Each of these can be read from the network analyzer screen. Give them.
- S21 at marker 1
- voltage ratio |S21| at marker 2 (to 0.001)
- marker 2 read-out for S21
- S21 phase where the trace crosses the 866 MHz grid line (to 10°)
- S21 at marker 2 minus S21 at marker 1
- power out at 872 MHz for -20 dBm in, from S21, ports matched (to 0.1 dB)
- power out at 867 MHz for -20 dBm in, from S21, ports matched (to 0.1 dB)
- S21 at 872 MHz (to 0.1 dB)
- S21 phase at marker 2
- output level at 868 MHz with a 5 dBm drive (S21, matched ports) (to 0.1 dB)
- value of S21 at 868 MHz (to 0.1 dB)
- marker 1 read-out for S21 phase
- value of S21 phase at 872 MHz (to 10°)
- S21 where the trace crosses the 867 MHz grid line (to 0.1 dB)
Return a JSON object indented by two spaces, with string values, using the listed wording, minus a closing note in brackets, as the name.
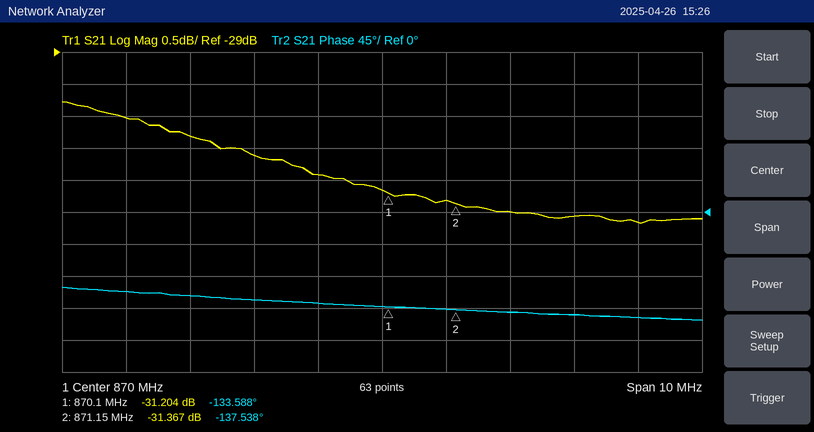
{
  "S21 at marker 1": "-31.204 dB",
  "voltage ratio |S21| at marker 2": "0.027",
  "marker 2 read-out for S21": "-31.367 dB",
  "S21 phase where the trace crosses the 866 MHz grid line": "-110°",
  "S21 at marker 2 minus S21 at marker 1": "-0.163 dB",
  "power out at 872 MHz for -20 dBm in, from S21, ports matched": "-51.5 dBm",
  "power out at 867 MHz for -20 dBm in, from S21, ports matched": "-50.3 dBm",
  "S21 at 872 MHz": "-31.5 dB",
  "S21 phase at marker 2": "-137.538°",
  "output level at 868 MHz with a 5 dBm drive (S21, matched ports)": "-25.6 dBm",
  "value of S21 at 868 MHz": "-30.6 dB",
  "marker 1 read-out for S21 phase": "-133.588°",
  "value of S21 phase at 872 MHz": "-140°",
  "S21 where the trace crosses the 867 MHz grid line": "-30.3 dB"
}
